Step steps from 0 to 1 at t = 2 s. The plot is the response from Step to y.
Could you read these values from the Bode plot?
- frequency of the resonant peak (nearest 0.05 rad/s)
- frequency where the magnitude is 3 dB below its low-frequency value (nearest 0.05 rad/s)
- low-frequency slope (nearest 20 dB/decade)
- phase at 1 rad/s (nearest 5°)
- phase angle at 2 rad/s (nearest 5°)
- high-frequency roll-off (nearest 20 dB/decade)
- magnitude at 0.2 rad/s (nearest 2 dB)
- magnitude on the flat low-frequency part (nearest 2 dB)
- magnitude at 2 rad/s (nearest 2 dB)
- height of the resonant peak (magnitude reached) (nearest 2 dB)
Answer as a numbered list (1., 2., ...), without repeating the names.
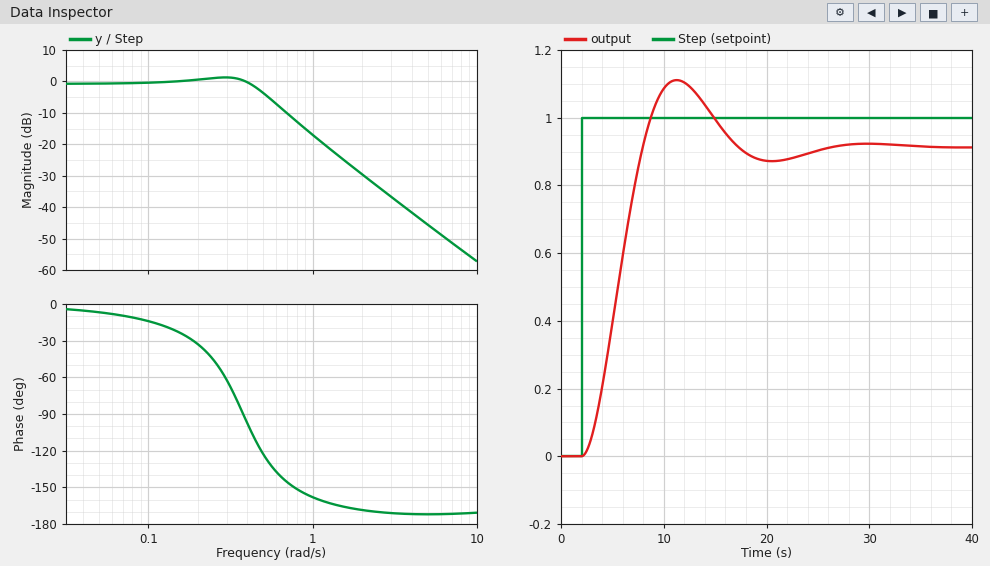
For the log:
1. 0.30 rad/s
2. 0.50 rad/s
3. 0 dB/decade
4. -160°
5. -170°
6. -40 dB/decade
7. 0 dB
8. 0 dB
9. -30 dB
10. 2 dB
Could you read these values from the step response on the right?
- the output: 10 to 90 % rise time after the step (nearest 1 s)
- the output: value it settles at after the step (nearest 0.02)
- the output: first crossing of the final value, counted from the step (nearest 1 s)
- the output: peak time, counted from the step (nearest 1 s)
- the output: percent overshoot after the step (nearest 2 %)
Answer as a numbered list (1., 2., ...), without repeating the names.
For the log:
1. 4 s
2. 0.92
3. 6 s
4. 9 s
5. 22 %
